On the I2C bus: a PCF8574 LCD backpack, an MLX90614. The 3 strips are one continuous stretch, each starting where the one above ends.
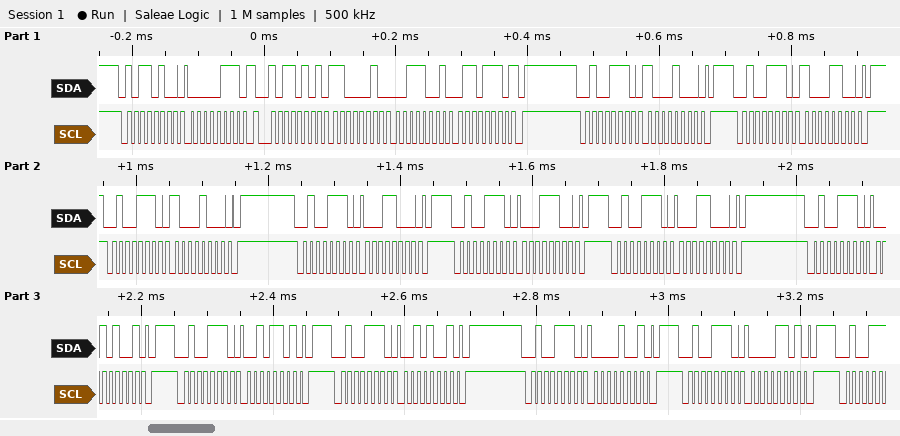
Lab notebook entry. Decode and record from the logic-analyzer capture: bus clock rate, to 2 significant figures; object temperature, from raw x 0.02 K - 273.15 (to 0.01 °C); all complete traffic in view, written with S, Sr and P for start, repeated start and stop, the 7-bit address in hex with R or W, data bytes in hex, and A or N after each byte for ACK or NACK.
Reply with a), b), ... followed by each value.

a) 100 kHz
b) 22.57 °C
c) S 5AW A 07 A Sr 5AR A C2 A 39 A 6E N P S 27W A 88 A P S 27W A 8C A P S 27W A 88 A P S 27W A 18 A P S 27W A 1C A P S 27W A 18 A P S 27W A 29 A P S 27W A 2D A P S 27W A 29 A P S 27W A 09 A P S 27W A 0D A P
